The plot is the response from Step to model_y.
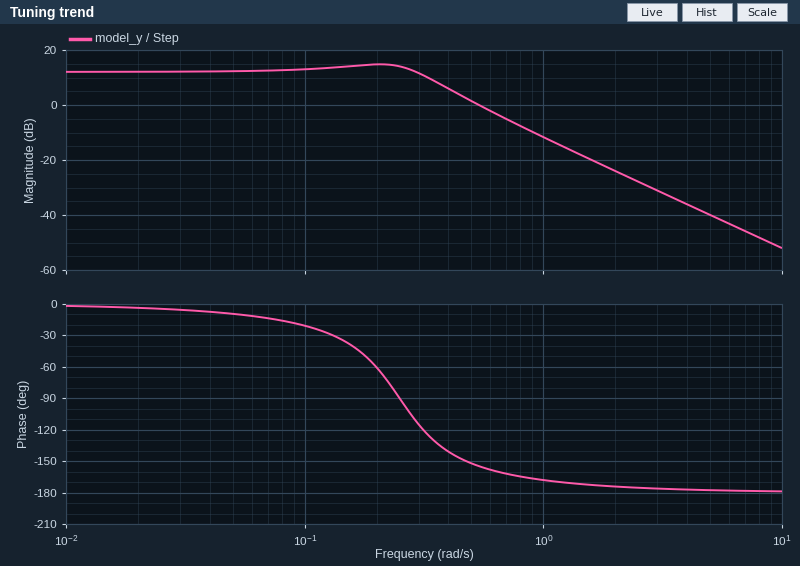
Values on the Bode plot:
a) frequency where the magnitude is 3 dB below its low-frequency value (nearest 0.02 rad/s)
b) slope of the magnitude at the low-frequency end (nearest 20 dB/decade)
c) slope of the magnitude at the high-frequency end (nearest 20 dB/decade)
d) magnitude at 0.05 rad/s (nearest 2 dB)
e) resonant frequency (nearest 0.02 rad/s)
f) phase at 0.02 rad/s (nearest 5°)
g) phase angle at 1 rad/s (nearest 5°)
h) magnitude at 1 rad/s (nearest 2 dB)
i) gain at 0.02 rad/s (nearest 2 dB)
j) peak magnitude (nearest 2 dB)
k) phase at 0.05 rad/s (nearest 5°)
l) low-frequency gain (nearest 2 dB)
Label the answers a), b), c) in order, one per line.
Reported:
a) 0.34 rad/s
b) 0 dB/decade
c) -40 dB/decade
d) 12 dB
e) 0.20 rad/s
f) -5°
g) -170°
h) -12 dB
i) 12 dB
j) 14 dB
k) -10°
l) 12 dB
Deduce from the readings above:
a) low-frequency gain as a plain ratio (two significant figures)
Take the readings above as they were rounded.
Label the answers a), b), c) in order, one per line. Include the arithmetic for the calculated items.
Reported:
a) 10^(12 / 20) = 4.0
